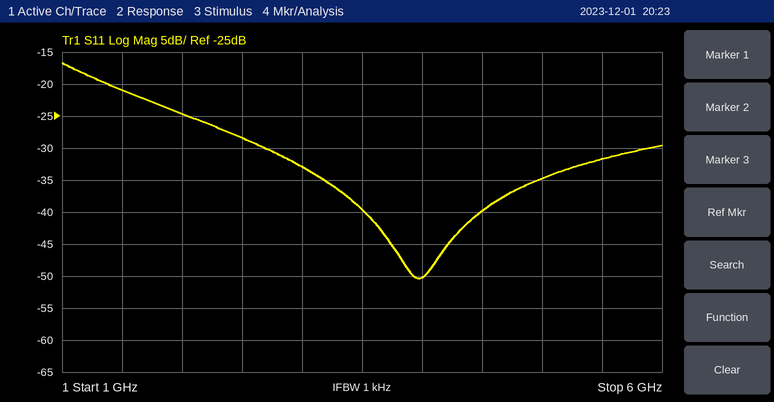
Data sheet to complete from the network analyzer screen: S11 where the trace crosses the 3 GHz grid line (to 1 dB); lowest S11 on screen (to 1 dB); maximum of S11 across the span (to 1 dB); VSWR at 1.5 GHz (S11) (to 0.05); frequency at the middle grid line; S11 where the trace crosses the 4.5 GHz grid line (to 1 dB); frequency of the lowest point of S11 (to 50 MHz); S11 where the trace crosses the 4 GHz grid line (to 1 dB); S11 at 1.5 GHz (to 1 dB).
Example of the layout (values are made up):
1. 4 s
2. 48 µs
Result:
1. -33 dB
2. -50 dB
3. -17 dB
4. 1.20
5. 3.5 GHz
6. -40 dB
7. 3.95 GHz
8. -50 dB
9. -21 dB
